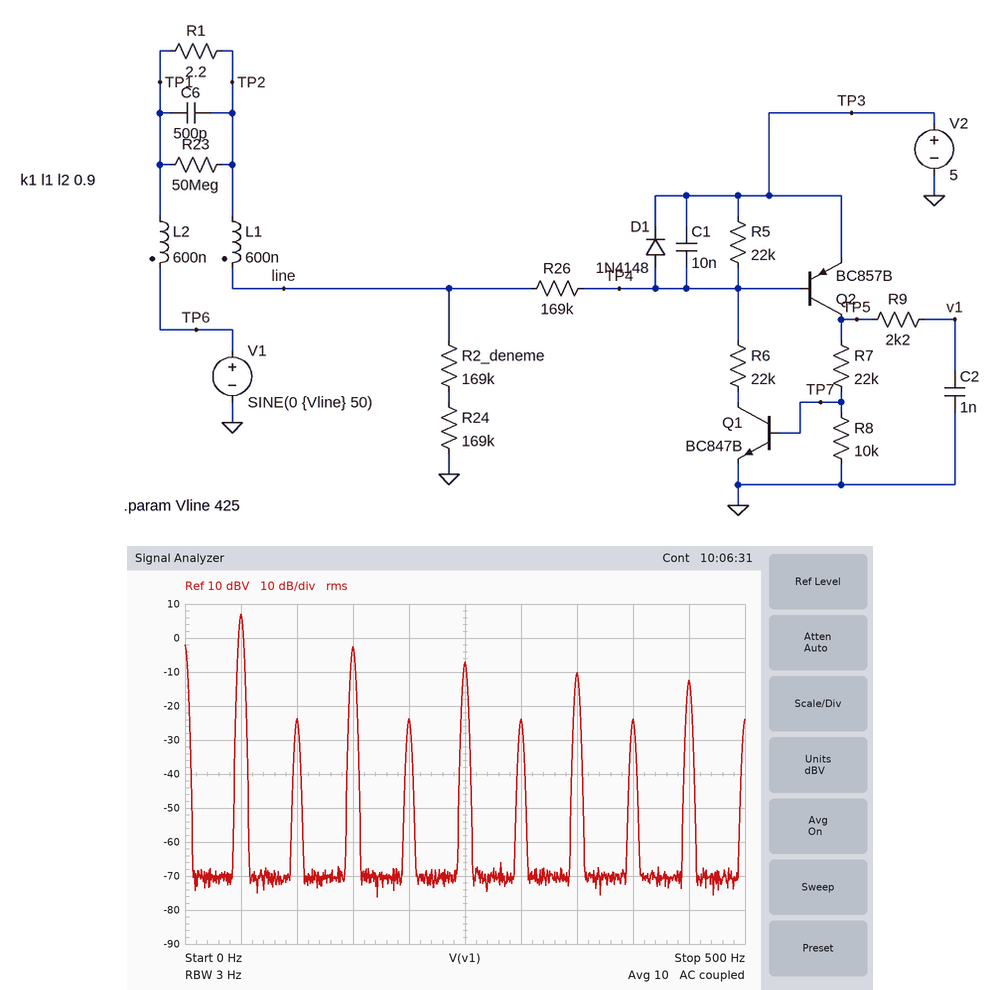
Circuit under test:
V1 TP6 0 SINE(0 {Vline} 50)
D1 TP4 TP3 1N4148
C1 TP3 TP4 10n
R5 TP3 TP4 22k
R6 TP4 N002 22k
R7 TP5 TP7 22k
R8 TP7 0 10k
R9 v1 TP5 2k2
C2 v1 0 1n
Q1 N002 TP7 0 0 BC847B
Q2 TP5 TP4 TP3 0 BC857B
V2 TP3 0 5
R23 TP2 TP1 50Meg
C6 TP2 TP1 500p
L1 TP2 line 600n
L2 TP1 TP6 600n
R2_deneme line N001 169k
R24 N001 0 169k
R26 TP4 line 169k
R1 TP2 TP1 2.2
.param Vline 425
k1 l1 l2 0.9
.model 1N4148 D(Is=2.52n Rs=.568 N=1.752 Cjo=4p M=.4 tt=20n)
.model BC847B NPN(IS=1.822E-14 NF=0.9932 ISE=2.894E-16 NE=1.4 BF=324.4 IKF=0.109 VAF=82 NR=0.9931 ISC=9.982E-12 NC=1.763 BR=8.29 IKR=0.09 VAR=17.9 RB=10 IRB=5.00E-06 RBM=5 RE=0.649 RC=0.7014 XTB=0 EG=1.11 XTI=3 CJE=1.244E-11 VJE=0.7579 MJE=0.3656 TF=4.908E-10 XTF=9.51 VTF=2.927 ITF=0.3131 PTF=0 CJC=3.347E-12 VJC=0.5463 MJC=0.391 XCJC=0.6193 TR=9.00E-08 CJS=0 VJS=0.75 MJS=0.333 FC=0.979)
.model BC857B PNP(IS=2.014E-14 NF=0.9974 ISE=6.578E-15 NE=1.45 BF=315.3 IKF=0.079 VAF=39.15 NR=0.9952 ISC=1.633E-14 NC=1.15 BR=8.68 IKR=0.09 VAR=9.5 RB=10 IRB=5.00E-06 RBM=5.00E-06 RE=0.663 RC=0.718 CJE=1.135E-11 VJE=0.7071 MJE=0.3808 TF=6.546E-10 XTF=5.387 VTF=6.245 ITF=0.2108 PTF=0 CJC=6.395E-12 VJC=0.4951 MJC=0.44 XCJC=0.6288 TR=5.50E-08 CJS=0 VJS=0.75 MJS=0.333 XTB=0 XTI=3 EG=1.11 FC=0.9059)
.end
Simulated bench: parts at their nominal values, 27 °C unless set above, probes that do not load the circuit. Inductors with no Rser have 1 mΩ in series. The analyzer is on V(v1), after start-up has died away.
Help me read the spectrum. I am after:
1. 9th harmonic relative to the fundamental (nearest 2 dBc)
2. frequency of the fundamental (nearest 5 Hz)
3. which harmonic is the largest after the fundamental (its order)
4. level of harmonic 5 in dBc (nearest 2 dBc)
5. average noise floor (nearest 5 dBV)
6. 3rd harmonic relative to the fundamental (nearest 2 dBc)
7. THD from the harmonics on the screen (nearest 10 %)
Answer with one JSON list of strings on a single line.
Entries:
["-20 dBc", "50 Hz", "3", "-14 dBc", "-70 dBV", "-10 dBc", "40 %"]
